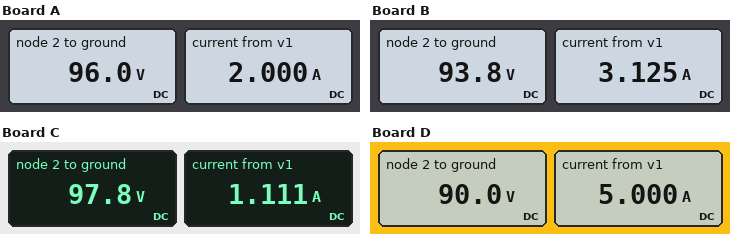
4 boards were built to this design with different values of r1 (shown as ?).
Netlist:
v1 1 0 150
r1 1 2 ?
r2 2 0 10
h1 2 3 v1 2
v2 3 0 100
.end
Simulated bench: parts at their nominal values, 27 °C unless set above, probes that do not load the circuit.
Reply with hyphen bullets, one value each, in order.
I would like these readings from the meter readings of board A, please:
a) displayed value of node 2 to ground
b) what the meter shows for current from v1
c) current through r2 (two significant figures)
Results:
- 96.0 V
- 2.000 A
- 9.6 A
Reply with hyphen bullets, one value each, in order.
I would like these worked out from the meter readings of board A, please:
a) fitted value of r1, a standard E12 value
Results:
- 27 Ω
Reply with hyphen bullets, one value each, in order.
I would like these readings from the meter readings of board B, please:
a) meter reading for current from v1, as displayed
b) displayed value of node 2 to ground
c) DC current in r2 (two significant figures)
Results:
- 3.125 A
- 93.8 V
- 9.4 A
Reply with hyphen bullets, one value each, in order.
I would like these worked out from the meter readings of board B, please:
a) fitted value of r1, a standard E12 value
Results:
- 18 Ω
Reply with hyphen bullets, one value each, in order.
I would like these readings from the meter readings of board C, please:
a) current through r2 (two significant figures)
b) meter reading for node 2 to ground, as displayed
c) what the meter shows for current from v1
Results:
- 9.8 A
- 97.8 V
- 1.111 A
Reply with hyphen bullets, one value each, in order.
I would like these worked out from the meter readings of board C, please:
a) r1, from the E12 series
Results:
- 47 Ω
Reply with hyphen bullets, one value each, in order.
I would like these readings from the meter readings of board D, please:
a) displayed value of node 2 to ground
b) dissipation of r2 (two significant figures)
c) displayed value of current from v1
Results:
- 90.0 V
- 810 W
- 5.000 A
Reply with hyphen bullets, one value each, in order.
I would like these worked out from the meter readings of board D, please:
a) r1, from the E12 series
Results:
- 12 Ω
